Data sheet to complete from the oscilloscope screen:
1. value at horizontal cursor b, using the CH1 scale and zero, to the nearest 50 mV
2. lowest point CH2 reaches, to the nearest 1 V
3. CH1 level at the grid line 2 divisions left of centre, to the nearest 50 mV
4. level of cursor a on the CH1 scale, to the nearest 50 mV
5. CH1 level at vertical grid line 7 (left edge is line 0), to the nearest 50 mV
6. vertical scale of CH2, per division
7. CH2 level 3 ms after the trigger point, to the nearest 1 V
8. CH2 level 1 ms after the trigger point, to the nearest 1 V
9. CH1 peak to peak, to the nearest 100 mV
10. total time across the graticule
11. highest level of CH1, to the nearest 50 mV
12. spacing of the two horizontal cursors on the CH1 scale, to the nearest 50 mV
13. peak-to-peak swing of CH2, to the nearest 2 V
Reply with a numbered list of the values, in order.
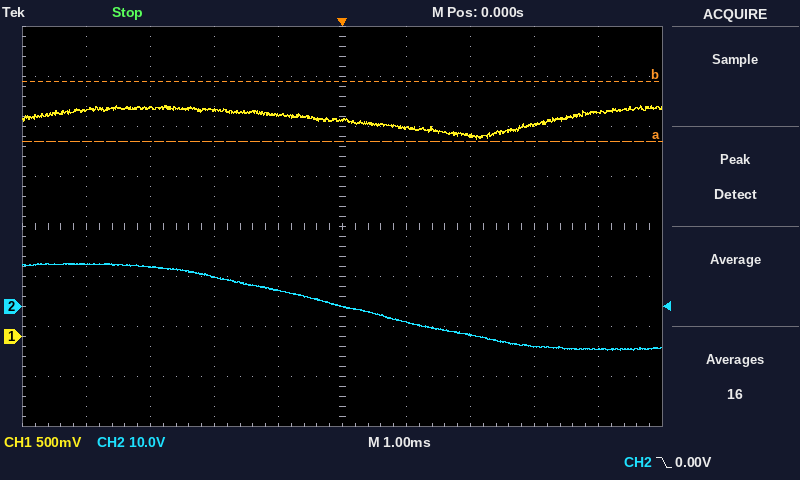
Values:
1. 2.55 V
2. -9 V
3. 2.25 V
4. 1.95 V
5. 2.00 V
6. 10 V
7. -8 V
8. -3 V
9. 300 mV
10. 10 ms
11. 2.30 V
12. 600 mV
13. 18 V
